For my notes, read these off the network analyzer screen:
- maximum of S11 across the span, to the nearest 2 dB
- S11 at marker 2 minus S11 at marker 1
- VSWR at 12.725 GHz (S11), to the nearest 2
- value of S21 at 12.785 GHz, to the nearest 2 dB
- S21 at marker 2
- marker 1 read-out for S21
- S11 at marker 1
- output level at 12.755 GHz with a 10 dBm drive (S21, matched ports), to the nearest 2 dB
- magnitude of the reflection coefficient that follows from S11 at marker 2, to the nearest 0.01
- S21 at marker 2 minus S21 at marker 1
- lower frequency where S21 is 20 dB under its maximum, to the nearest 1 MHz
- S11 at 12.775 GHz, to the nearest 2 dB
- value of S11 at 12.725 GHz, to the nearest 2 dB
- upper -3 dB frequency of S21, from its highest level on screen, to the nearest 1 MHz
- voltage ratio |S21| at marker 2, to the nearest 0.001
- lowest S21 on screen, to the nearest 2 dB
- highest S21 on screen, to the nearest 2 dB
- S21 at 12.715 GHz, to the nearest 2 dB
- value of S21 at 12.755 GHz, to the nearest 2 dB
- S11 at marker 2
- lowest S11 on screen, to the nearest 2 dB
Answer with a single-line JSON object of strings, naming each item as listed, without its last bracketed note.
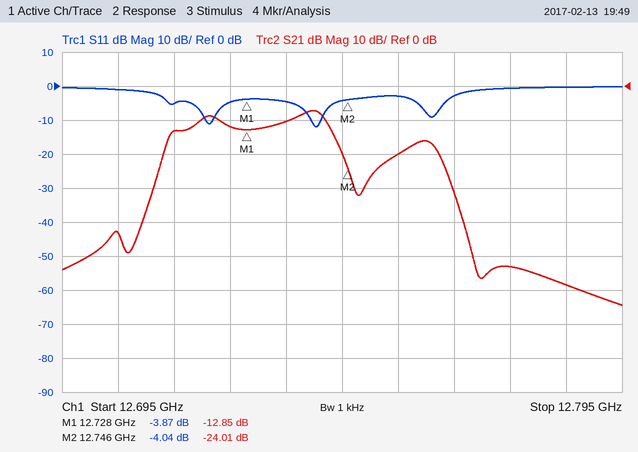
{"maximum of S11 across the span, to the nearest 2 dB": "0 dB", "S11 at marker 2 minus S11 at marker 1": "-0.17 dB", "VSWR at 12.725 GHz (S11), to the nearest 2": "4", "value of S21 at 12.785 GHz, to the nearest 2 dB": "-58 dB", "S21 at marker 2": "-24.01 dB", "marker 1 read-out for S21": "-12.85 dB", "S11 at marker 1": "-3.87 dB", "output level at 12.755 GHz with a 10 dBm drive (S21, matched ports), to the nearest 2 dB": "-10 dBm", "magnitude of the reflection coefficient that follows from S11 at marker 2, to the nearest 0.01": "0.63", "S21 at marker 2 minus S21 at marker 1": "-11.16 dB", "lower frequency where S21 is 20 dB under its maximum, to the nearest 1 MHz": "12.712 GHz", "S11 at 12.775 GHz, to the nearest 2 dB": "0 dB", "value of S11 at 12.725 GHz, to the nearest 2 dB": "-4 dB", "upper -3 dB frequency of S21, from its highest level on screen, to the nearest 1 MHz": "12.742 GHz", "voltage ratio |S21| at marker 2, to the nearest 0.001": "0.063", "lowest S21 on screen, to the nearest 2 dB": "-64 dB", "highest S21 on screen, to the nearest 2 dB": "-8 dB", "S21 at 12.715 GHz, to the nearest 2 dB": "-14 dB", "value of S21 at 12.755 GHz, to the nearest 2 dB": "-20 dB", "S11 at marker 2": "-4.04 dB", "lowest S11 on screen, to the nearest 2 dB": "-12 dB"}
